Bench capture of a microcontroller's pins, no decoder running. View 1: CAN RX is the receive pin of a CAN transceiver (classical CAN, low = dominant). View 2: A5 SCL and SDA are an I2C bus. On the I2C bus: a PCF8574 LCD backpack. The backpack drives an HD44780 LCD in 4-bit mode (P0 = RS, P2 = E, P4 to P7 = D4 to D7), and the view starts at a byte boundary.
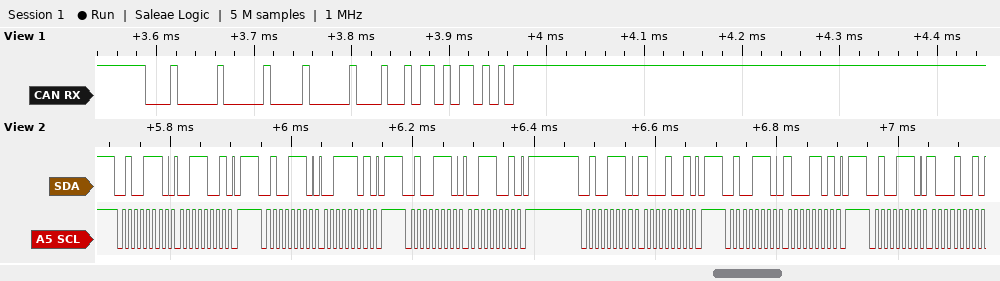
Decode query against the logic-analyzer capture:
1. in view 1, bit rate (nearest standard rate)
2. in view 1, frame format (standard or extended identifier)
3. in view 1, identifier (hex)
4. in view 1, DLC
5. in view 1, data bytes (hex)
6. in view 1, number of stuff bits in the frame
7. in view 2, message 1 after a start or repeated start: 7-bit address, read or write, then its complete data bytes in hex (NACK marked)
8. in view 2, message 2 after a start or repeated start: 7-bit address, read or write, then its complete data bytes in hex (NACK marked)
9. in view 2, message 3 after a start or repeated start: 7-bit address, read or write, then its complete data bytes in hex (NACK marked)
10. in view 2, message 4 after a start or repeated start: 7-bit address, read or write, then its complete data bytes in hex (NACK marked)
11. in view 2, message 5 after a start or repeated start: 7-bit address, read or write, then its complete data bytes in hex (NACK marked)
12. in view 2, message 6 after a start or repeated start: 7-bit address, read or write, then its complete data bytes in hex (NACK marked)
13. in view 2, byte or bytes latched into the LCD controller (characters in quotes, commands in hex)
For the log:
125 kbit/s
standard
0x100
1
00
3
0x27 write: 39
0x27 write: 3D
0x27 write: 39
0x27 write: 89
0x27 write: 8D
0x27 write: 89
'8'
